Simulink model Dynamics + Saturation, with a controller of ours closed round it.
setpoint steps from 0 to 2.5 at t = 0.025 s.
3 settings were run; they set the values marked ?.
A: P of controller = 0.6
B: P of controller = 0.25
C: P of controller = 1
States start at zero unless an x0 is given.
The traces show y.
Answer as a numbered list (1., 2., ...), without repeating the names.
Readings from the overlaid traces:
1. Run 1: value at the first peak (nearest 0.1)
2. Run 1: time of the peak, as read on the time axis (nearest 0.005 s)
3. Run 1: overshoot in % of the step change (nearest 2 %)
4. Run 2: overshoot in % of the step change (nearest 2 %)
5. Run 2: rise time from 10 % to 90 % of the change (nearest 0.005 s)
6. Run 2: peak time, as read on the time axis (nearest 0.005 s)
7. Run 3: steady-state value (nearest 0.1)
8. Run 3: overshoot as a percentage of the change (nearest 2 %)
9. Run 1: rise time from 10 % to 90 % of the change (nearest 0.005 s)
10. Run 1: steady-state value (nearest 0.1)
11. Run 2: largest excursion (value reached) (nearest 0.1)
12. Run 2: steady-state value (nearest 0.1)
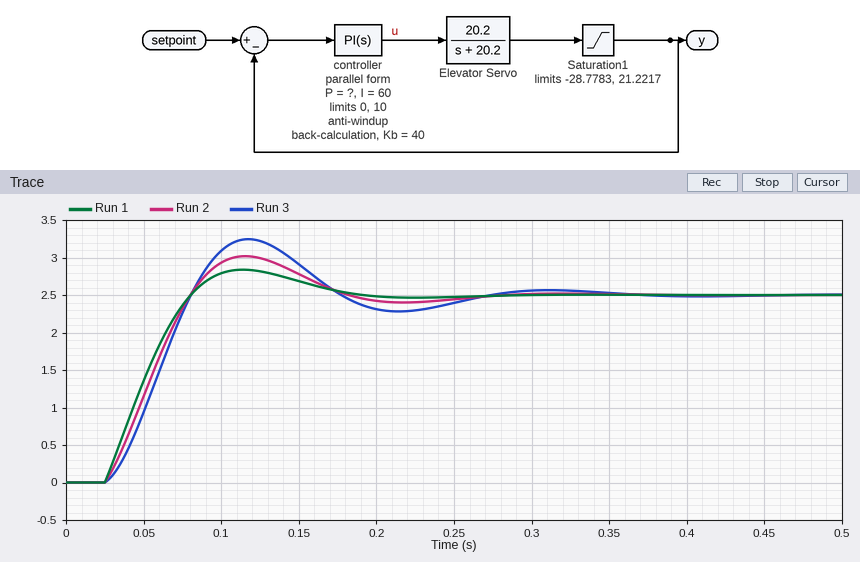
1. 2.8
2. 0.115 s
3. 14 %
4. 20 %
5. 0.040 s
6. 0.115 s
7. 2.5
8. 30 %
9. 0.040 s
10. 2.5
11. 3.0
12. 2.5
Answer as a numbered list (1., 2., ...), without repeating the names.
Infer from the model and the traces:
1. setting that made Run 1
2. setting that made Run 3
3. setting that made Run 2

1. C
2. B
3. A
